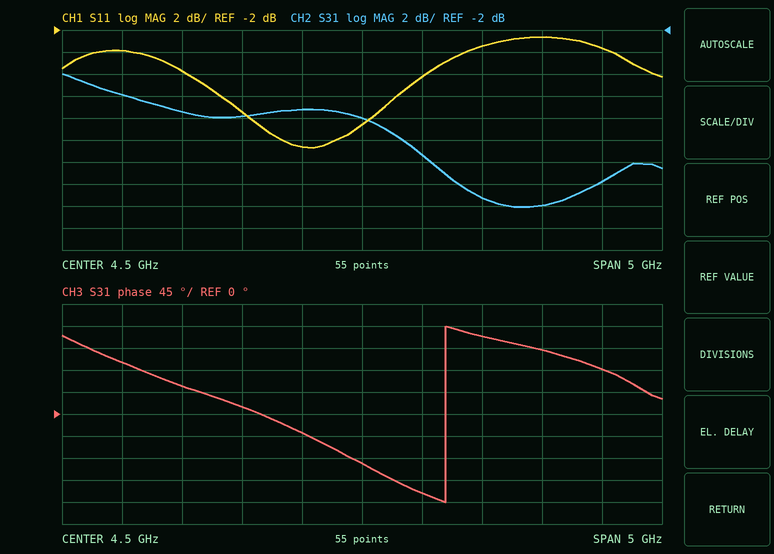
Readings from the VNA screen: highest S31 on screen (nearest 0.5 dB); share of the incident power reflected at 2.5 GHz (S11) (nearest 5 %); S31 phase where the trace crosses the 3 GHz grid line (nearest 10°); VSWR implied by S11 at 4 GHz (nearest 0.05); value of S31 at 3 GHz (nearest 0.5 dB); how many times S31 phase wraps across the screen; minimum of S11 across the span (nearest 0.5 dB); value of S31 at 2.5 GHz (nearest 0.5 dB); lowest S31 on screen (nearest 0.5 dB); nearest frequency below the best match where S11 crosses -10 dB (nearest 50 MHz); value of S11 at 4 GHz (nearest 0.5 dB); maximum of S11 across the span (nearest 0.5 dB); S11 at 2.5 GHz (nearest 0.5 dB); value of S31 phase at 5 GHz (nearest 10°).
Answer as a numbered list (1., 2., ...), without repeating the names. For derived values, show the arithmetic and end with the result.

1. -6.0 dB
2. 10^(-4/10) ≈ 40 %
3. 60°
4. |Γ| = 10^(-12.5/20) = 0.2371; VSWR = (1 + 0.2371)/(1 − 0.2371) ≈ 1.62, so 1.60 to the nearest 0.05
5. -9.5 dB
6. 1
7. -12.5 dB
8. -8.0 dB
9. -18.0 dB
10. 3.55 GHz
11. -12.5 dB
12. -2.5 dB
13. -4.0 dB
14. -160°
